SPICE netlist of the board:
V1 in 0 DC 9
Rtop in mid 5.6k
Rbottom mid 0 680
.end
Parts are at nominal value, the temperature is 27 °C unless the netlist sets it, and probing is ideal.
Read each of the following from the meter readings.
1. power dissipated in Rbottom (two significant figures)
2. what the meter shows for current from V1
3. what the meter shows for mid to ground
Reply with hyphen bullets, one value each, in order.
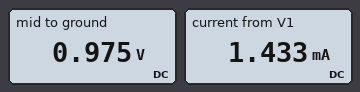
- 1.4 mW
- 1.433 mA
- 0.975 V
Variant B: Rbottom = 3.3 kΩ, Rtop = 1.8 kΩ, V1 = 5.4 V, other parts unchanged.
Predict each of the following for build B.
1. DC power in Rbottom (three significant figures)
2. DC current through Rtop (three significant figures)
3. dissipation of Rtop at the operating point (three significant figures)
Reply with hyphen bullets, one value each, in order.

- 3.70 mW
- 1.06 mA
- 2.02 mW
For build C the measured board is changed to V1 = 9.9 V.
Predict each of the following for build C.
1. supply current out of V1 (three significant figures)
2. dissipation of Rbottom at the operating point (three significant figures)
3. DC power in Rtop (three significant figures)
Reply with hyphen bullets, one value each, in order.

- 1.58 mA
- 1.69 mW
- 13.9 mW
